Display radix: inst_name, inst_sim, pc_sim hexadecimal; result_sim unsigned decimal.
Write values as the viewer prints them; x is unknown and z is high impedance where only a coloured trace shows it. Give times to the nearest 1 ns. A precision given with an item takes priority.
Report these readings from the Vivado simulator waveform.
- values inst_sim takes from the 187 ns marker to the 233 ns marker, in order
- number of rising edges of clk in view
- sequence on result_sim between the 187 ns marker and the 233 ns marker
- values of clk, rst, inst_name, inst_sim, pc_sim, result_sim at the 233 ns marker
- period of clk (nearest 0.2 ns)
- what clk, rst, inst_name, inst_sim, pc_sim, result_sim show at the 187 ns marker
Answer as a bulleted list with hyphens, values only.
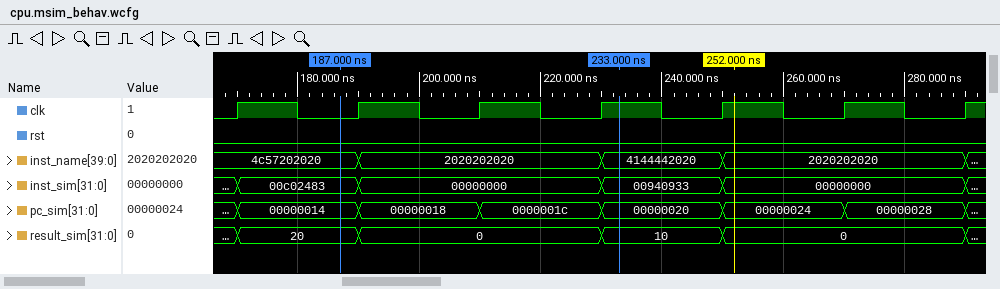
- 00c02483, 00000000, 00940933
- 7
- 20, 0, 10
- clk=1, rst=0, inst_name=4144442020, inst_sim=00940933, pc_sim=00000020, result_sim=10
- 20 ns
- clk=0, rst=0, inst_name=4c57202020, inst_sim=00c02483, pc_sim=00000014, result_sim=20
